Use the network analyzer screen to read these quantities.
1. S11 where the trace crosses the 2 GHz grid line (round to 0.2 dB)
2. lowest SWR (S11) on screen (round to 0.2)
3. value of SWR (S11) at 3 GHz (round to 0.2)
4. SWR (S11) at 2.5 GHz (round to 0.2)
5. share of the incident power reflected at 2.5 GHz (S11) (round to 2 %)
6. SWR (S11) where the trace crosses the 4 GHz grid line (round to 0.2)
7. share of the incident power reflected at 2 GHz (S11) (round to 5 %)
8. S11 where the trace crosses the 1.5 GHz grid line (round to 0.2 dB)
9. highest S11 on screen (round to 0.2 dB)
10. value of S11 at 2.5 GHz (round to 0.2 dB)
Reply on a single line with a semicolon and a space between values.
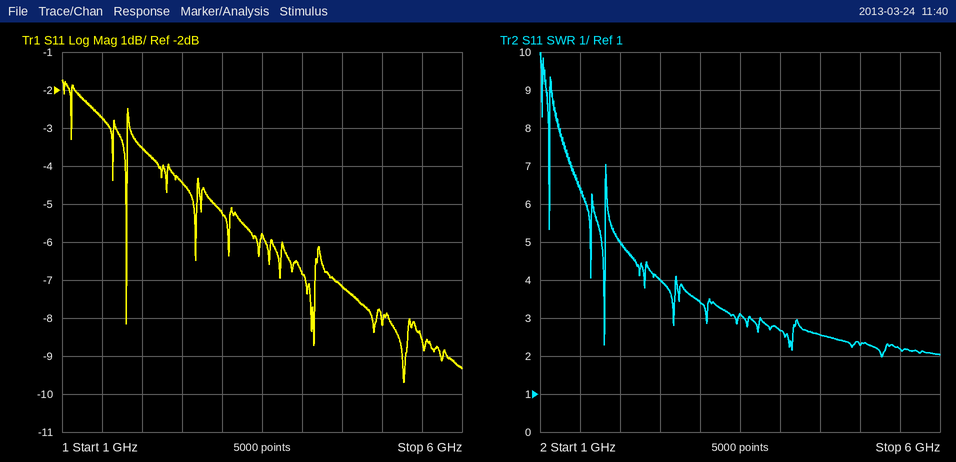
-3.6 dB; 2.0; 3.4; 4.0; 36 %; 2.6; 45 %; -2.8 dB; -1.8 dB; -4.4 dB
